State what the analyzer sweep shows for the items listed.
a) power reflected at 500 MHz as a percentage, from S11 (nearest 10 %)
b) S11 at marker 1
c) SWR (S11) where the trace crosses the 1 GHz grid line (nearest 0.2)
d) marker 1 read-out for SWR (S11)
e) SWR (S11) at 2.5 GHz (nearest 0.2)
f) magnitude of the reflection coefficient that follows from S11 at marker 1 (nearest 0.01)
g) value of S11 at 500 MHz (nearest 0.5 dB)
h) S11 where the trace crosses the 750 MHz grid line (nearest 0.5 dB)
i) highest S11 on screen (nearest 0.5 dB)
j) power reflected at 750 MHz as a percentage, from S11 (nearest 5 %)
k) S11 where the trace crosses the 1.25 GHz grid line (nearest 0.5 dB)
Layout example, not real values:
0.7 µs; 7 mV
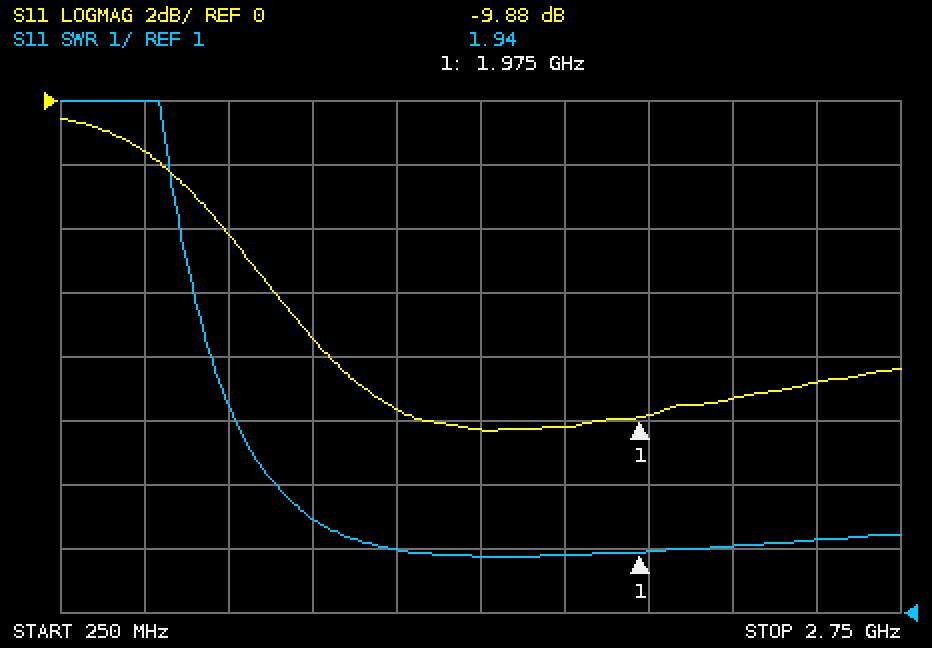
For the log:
70 %; -9.88 dB; 2.4; 1.94; 2.2; 0.32; -1.5 dB; -4.0 dB; -0.5 dB; 40 %; -9.5 dB
